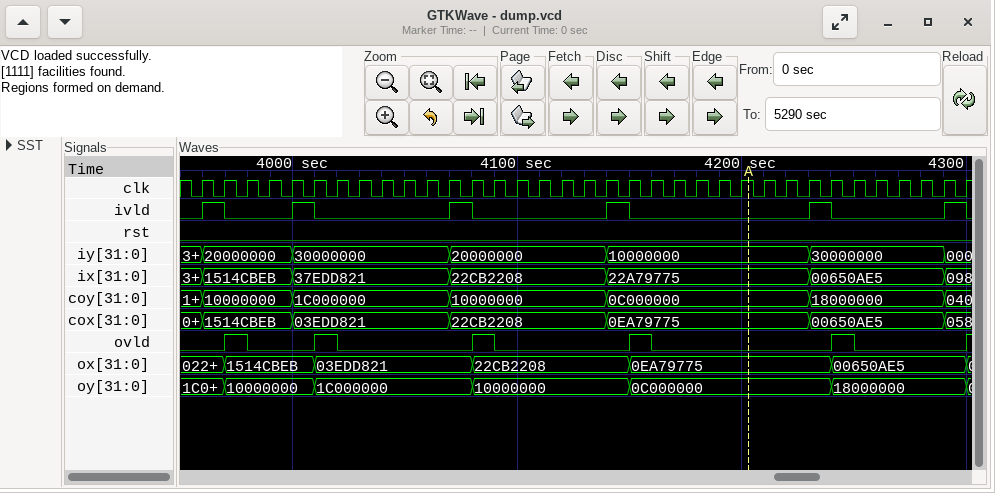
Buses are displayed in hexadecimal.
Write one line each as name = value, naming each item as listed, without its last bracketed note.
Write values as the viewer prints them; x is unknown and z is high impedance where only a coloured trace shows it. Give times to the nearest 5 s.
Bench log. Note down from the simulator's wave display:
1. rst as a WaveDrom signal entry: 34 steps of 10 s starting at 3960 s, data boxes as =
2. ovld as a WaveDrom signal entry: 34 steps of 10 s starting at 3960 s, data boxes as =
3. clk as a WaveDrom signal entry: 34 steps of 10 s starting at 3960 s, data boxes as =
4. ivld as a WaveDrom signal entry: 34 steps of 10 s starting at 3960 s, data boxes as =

rst as a WaveDrom signal entry: 34 steps of 10 s starting at 3960 s, data boxes as = = {name: 'rst', wave: '0.................................'}
ovld as a WaveDrom signal entry: 34 steps of 10 s starting at 3960 s, data boxes as = = {name: 'ovld', wave: '010..10.....10.....10.......10....'}
clk as a WaveDrom signal entry: 34 steps of 10 s starting at 3960 s, data boxes as = = {name: 'clk', wave: 'p.................................'}
ivld as a WaveDrom signal entry: 34 steps of 10 s starting at 3960 s, data boxes as = = {name: 'ivld', wave: '10..10.....10.....10.......10....1'}
